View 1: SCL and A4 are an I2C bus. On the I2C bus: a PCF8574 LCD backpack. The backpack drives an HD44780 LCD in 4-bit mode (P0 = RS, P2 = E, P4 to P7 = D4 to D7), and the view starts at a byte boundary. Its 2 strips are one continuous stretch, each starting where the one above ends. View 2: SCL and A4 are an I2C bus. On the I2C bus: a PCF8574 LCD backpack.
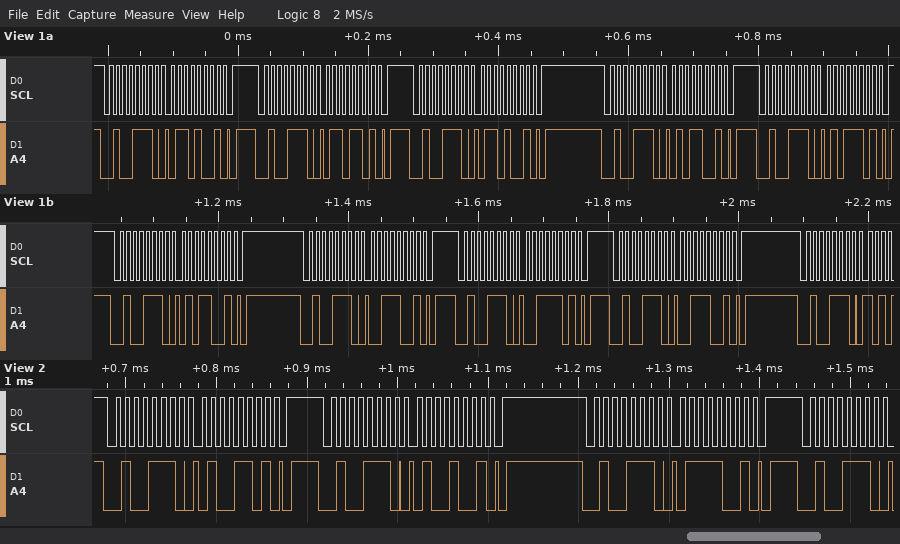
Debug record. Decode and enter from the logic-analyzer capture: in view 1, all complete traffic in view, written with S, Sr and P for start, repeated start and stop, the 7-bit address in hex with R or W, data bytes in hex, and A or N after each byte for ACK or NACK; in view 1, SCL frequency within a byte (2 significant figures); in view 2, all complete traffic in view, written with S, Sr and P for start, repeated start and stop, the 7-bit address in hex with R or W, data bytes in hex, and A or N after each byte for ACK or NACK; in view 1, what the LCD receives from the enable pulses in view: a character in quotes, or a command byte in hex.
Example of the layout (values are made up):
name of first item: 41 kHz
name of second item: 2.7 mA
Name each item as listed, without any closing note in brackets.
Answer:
in view 1, all complete traffic in view, written with S, Sr and P for start, repeated start and stop, the 7-bit address in hex with R or W, data bytes in hex, and A or N after each byte for ACK or NACK: S 27W A 69 A P S 27W A 6D A P S 27W A 69 A P S 27W A 59 A P S 27W A 5D A P S 27W A 59 A P S 27W A 39 A P S 27W A 3D A P S 27W A 39 A P S 27W A
in view 1, SCL frequency within a byte: 100 kHz
in view 2, all complete traffic in view, written with S, Sr and P for start, repeated start and stop, the 7-bit address in hex with R or W, data bytes in hex, and A or N after each byte for ACK or NACK: S 27W A 4D A P S 27W A 49 A P S 27W A 79 A P S 27W A
in view 1, what the LCD receives from the enable pulses in view: a character in quotes, or a command byte in hex: 'e'
